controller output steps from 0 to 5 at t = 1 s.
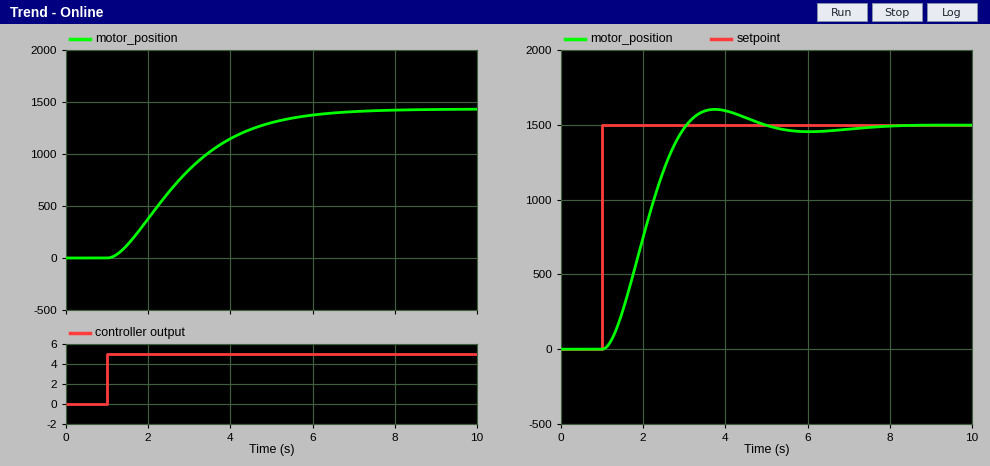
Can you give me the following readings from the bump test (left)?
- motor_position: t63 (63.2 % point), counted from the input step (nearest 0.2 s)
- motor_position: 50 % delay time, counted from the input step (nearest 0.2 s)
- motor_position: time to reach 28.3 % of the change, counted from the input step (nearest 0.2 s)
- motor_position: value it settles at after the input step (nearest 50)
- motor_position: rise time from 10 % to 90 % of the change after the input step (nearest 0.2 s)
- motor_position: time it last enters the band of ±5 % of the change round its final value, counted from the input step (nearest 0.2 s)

2.2 s
1.6 s
1.0 s
1450
3.4 s
4.8 s
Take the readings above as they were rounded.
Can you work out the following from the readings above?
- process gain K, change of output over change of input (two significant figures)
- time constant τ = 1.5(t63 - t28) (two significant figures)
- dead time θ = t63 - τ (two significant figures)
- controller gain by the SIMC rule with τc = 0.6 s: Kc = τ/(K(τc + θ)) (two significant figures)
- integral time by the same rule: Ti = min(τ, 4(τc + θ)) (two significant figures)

290
1.8 s
0.40 s
0.0062
1.8 s
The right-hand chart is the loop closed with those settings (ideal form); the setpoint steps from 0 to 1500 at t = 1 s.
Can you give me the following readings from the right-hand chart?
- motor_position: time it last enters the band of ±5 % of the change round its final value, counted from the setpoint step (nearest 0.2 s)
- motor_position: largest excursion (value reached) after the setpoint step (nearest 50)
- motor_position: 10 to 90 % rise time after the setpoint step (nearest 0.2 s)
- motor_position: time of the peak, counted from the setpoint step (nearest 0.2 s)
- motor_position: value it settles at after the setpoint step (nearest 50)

3.2 s
1600
1.4 s
2.8 s
1500
